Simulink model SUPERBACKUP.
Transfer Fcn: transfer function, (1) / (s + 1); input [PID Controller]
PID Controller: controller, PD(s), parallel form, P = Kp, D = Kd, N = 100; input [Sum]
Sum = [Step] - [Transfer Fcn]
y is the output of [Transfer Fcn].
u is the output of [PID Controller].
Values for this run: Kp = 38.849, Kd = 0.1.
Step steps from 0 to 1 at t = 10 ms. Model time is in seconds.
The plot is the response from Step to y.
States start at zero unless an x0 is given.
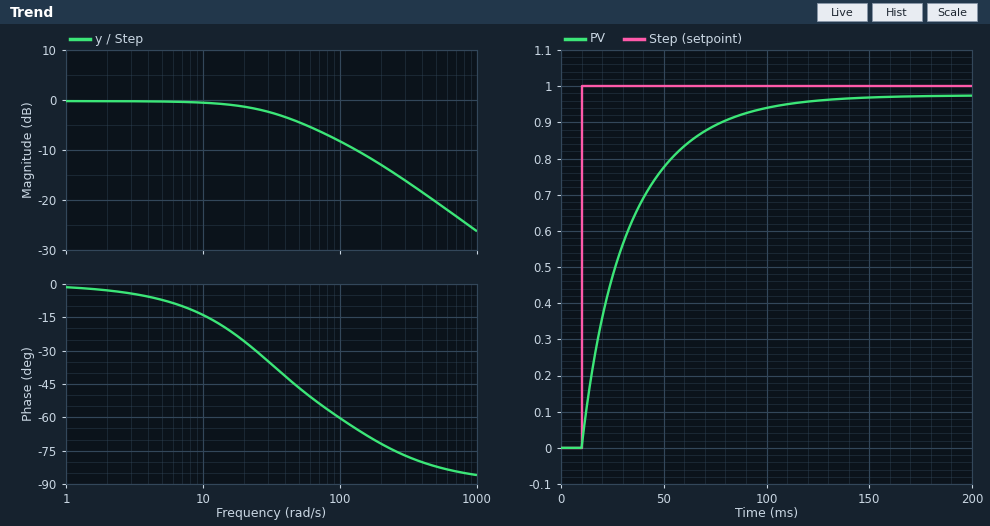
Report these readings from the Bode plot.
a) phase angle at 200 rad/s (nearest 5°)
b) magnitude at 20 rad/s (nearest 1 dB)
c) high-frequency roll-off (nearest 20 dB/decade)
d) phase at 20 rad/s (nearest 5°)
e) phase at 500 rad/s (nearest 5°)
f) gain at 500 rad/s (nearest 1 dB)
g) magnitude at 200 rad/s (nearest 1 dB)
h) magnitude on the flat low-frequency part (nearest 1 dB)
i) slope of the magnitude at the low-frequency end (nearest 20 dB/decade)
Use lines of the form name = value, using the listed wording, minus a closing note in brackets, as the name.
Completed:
phase angle at 200 rad/s = -70°
magnitude at 20 rad/s = -1 dB
high-frequency roll-off = -20 dB/decade
phase at 20 rad/s = -25°
phase at 500 rad/s = -80°
gain at 500 rad/s = -20 dB
magnitude at 200 rad/s = -13 dB
magnitude on the flat low-frequency part = 0 dB
slope of the magnitude at the low-frequency end = 0 dB/decade
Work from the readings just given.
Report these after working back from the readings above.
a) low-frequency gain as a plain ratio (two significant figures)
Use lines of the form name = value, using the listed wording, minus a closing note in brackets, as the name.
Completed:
low-frequency gain as a plain ratio = 1.0
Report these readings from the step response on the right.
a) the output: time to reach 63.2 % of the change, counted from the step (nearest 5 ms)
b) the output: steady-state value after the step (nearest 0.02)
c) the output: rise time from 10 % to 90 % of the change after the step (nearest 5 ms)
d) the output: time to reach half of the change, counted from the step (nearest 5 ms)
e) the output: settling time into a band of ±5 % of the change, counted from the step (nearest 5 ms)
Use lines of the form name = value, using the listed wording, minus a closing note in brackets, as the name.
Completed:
the output: time to reach 63.2 % of the change, counted from the step = 25 ms
the output: steady-state value after the step = 0.98
the output: rise time from 10 % to 90 % of the change after the step = 60 ms
the output: time to reach half of the change, counted from the step = 15 ms
the output: settling time into a band of ±5 % of the change, counted from the step = 80 ms
